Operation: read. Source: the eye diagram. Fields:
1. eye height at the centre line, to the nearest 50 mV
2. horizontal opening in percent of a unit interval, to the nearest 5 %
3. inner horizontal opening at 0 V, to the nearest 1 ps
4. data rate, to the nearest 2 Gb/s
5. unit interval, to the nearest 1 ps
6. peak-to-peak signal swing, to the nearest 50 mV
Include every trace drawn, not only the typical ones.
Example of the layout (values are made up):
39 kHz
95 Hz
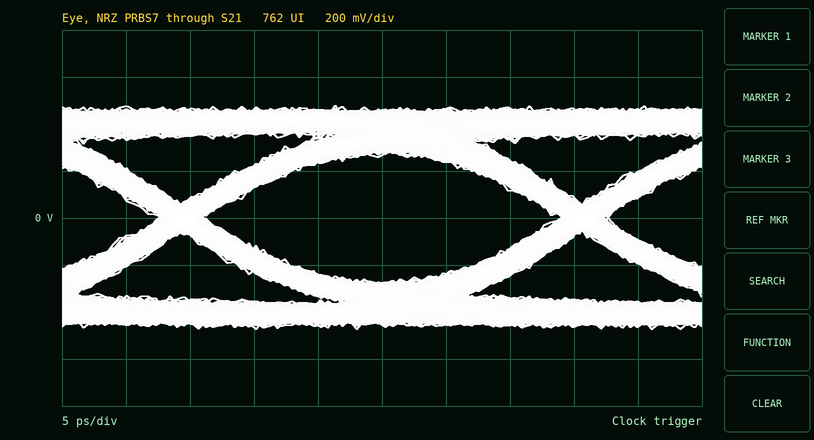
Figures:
550 mV
90 %
28 ps
32 Gb/s
31 ps
950 mV
